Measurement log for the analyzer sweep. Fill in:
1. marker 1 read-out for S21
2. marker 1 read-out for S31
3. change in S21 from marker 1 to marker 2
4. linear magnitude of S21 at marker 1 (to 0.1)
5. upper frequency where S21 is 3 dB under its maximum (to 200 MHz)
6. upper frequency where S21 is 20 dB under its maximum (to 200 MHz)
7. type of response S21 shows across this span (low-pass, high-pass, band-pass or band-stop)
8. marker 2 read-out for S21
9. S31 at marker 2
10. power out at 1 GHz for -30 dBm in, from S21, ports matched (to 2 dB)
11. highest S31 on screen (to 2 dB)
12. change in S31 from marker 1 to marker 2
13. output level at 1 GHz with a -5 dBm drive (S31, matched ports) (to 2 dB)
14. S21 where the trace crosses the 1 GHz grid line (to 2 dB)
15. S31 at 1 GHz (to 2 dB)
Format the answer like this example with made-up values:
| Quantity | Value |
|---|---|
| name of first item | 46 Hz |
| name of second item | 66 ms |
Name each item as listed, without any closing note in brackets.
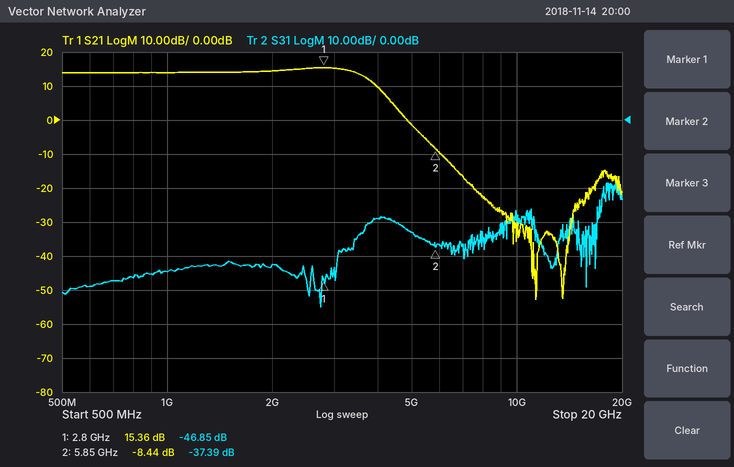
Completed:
| Quantity | Value |
|---|---|
| marker 1 read-out for S21 | 15.36 dB |
| marker 1 read-out for S31 | -46.85 dB |
| change in S21 from marker 1 to marker 2 | -23.80 dB |
| linear magnitude of S21 at marker 1 | 5.9 |
| upper frequency where S21 is 3 dB under its maximum | 3.8 GHz |
| upper frequency where S21 is 20 dB under its maximum | 5.4 GHz |
| type of response S21 shows across this span | low-pass |
| marker 2 read-out for S21 | -8.44 dB |
| S31 at marker 2 | -37.39 dB |
| power out at 1 GHz for -30 dBm in, from S21, ports matched | -16 dBm |
| highest S31 on screen | -18 dB |
| change in S31 from marker 1 to marker 2 | 9.46 dB |
| output level at 1 GHz with a -5 dBm drive (S31, matched ports) | -50 dBm |
| S21 where the trace crosses the 1 GHz grid line | 14 dB |
| S31 at 1 GHz | -44 dB |
